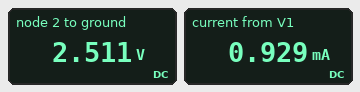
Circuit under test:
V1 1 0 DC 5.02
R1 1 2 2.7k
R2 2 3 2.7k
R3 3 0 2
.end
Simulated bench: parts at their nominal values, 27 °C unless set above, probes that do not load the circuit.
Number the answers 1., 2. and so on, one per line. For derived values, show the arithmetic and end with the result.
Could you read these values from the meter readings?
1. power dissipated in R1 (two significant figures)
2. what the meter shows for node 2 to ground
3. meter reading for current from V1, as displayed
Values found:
1. (5.02 V - 2.511 V)^2 / 2.7 kΩ = 2.3 mW
2. 2.511 V
3. 0.929 mA
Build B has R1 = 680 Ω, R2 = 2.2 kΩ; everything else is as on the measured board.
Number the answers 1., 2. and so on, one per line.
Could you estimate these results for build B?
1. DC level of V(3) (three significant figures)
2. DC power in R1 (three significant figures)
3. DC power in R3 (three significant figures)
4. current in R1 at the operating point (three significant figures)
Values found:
1. 3.48 mV
2. 2.06 mW
3. 6.07 µW
4. 1.74 mA
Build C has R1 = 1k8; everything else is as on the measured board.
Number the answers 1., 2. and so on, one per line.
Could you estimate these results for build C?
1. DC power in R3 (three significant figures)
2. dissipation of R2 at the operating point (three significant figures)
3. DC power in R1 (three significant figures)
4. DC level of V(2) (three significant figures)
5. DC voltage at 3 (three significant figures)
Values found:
1. 2.49 µW
2. 3.36 mW
3. 2.24 mW
4. 3.01 V
5. 2.23 mV
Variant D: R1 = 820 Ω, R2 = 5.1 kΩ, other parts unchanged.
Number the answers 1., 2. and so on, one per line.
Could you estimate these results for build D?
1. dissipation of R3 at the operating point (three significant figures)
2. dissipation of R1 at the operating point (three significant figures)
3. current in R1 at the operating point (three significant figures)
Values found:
1. 1.44 µW
2. 589 µW
3. 848 µA
